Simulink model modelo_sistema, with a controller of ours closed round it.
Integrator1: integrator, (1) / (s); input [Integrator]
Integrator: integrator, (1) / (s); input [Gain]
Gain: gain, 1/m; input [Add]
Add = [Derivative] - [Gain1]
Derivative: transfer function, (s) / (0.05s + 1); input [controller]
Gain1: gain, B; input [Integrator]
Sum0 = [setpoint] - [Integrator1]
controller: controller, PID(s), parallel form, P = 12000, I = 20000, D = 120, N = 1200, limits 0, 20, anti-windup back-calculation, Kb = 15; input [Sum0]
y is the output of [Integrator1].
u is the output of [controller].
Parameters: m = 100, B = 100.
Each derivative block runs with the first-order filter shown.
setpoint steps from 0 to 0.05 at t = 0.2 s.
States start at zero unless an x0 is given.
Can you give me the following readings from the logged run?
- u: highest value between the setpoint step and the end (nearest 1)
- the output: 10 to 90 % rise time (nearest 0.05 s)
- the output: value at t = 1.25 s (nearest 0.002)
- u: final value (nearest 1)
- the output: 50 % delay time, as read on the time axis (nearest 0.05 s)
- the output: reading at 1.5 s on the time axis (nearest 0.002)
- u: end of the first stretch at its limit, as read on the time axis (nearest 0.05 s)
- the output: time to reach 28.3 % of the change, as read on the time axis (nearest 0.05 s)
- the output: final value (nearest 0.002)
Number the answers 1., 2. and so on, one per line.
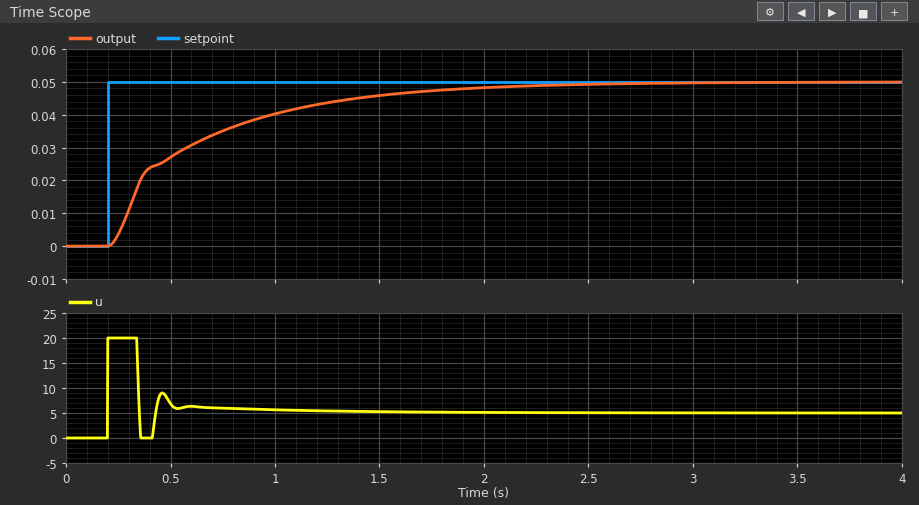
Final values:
1. 20
2. 1.15 s
3. 0.044
4. 5
5. 0.45 s
6. 0.046
7. 0.35 s
8. 0.30 s
9. 0.050
